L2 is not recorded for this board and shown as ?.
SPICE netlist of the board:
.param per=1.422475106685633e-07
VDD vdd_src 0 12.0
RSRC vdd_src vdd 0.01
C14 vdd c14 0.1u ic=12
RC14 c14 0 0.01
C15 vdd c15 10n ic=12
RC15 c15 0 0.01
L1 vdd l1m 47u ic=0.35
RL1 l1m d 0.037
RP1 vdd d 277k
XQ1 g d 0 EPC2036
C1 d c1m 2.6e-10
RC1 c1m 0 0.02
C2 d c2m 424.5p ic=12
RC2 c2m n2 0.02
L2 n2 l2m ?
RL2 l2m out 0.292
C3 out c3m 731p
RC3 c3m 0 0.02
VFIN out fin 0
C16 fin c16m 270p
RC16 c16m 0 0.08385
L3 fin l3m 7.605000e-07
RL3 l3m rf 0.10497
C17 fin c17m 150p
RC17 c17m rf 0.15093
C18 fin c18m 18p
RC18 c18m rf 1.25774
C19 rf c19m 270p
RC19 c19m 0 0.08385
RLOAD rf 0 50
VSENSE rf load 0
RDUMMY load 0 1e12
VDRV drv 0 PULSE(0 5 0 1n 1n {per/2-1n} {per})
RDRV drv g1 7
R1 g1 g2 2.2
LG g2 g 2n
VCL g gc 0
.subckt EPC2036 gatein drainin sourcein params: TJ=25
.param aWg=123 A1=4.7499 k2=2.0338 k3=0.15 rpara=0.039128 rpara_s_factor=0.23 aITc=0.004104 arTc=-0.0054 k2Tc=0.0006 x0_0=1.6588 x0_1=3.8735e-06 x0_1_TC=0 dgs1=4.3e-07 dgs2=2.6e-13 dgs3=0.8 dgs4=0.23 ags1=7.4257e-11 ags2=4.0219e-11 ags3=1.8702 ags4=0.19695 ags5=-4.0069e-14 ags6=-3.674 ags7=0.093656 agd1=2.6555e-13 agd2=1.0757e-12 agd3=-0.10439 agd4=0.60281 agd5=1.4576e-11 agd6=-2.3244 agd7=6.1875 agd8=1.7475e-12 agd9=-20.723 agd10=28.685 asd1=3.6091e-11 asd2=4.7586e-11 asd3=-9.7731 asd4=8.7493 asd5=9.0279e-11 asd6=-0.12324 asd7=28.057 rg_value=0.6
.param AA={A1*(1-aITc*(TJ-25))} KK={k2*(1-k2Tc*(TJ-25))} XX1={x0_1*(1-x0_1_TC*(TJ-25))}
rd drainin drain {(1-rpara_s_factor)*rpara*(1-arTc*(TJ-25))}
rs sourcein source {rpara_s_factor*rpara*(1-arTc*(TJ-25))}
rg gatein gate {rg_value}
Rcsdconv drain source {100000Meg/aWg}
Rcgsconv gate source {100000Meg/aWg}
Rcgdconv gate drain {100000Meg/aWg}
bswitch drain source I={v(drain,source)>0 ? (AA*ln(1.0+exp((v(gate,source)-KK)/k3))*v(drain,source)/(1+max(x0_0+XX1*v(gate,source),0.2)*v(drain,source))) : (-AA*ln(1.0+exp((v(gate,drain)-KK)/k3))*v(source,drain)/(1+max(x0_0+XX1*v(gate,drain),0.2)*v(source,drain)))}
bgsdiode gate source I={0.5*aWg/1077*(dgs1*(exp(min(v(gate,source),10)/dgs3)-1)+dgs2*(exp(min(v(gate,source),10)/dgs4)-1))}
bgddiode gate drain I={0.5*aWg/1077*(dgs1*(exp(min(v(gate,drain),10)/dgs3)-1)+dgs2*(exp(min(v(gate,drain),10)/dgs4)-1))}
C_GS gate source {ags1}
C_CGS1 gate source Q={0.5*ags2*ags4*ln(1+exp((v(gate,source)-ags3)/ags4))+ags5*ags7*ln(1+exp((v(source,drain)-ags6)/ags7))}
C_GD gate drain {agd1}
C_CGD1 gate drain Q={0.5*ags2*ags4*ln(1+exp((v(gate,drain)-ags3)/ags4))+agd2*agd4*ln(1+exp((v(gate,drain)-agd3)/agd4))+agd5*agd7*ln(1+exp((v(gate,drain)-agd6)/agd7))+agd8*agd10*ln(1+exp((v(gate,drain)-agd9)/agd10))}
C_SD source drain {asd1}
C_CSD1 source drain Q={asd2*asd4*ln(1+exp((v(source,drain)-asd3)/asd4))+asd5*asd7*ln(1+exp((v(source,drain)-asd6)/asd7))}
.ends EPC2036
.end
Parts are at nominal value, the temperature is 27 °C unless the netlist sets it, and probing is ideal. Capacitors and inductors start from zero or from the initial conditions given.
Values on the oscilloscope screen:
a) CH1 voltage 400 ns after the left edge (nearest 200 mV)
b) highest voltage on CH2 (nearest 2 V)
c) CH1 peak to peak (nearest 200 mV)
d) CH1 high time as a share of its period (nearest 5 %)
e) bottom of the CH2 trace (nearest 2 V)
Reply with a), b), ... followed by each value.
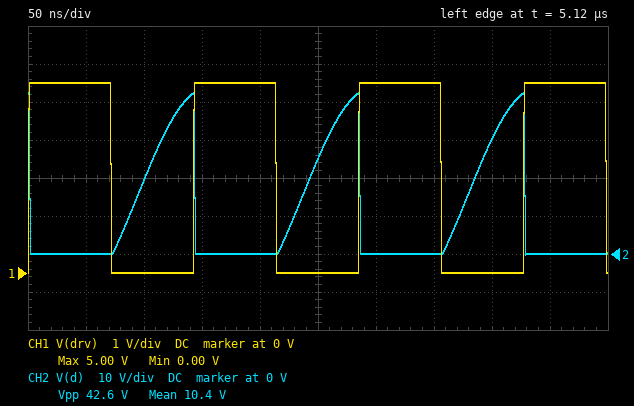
a) 0 V
b) 42 V
c) 5.0 V
d) 50 %
e) 0 V
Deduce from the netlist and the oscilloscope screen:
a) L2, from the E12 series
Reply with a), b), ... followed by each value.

a) 6.8 µH
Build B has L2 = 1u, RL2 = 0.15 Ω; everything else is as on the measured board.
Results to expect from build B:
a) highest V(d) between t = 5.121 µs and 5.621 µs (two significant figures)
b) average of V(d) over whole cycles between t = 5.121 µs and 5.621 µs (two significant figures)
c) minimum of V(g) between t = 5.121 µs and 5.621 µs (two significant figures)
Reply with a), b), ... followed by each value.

a) 67 V
b) 11 V
c) 5.6 mV
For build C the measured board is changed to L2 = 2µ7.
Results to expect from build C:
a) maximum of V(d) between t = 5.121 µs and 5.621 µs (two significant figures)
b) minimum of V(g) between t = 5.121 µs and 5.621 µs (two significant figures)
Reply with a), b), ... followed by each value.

a) 35 V
b) -25 mV
